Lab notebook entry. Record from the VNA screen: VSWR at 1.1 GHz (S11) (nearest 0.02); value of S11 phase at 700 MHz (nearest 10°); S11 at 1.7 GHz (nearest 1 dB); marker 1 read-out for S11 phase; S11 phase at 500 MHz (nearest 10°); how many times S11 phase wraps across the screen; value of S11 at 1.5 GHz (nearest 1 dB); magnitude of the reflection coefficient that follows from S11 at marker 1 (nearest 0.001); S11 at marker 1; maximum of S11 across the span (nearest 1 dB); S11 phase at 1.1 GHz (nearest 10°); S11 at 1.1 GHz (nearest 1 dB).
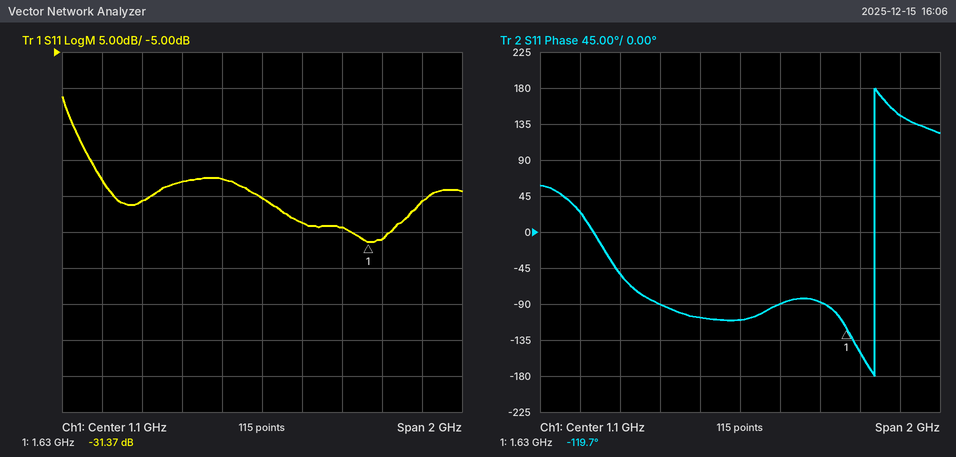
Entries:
1.12
-90°
-31 dB
-119.7°
-50°
1
-29 dB
0.027
-31.37 dB
-11 dB
-110°
-25 dB
